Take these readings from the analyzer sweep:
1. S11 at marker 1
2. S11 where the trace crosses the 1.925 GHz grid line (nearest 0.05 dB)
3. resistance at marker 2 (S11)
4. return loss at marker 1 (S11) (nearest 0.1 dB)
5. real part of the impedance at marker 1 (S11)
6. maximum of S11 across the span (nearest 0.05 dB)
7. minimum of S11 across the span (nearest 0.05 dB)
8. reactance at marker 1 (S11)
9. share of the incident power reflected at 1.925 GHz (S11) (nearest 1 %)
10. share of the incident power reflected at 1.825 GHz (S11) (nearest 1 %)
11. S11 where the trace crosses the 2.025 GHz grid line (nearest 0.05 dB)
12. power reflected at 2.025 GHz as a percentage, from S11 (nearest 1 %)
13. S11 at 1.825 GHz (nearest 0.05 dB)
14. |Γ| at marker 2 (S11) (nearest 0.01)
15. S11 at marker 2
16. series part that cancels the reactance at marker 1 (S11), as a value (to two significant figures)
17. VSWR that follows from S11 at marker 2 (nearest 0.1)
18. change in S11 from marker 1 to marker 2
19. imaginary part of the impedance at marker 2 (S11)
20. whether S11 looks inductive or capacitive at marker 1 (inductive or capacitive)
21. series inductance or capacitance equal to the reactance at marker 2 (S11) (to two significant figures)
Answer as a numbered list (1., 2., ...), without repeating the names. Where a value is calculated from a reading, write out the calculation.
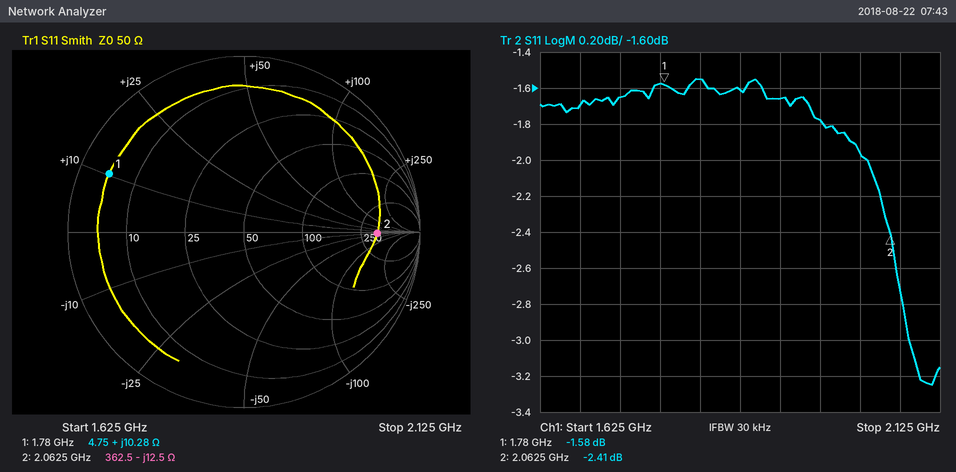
1. -1.58 dB
2. -1.65 dB
3. 362.5 Ω
4. 1.6 dB
5. 4.75 Ω
6. -1.55 dB
7. -3.25 dB
8. +10.28 Ω
9. 10^(-1.65/10) ≈ 68 %
10. 10^(-1.55/10) ≈ 70 %
11. -1.95 dB
12. 10^(-1.95/10) ≈ 64 %
13. -1.55 dB
14. 0.76
15. -2.41 dB
16. C = 1/(2π × 1.78 GHz × 10.28 Ω) ≈ 8.7 pF
17. (1 + 0.7577)/(1 − 0.7577) ≈ 7.3
18. -2.41 − (-1.58) = -0.83 dB
19. -12.5 Ω
20. inductive
21. C = 1/(2π × 2.0625 GHz × 12.5 Ω) ≈ 6.2 pF
